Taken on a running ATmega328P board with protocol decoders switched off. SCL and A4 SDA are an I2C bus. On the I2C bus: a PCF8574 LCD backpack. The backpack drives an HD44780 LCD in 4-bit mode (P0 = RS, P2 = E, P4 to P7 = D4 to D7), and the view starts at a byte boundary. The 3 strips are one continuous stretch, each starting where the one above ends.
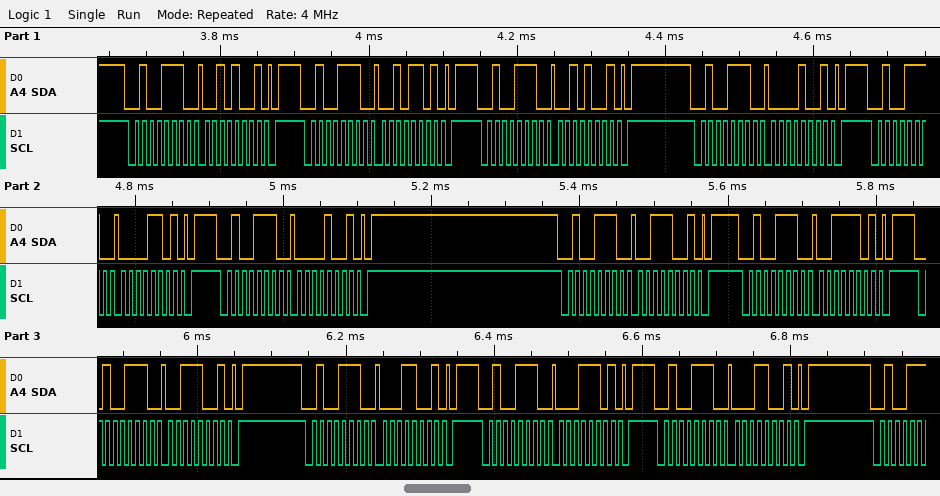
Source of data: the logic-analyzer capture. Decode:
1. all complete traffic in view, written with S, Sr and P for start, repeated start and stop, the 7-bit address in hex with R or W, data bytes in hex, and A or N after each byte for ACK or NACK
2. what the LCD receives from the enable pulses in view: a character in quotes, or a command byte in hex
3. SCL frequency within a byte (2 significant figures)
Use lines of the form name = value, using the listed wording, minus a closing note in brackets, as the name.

all complete traffic in view, written with S, Sr and P for start, repeated start and stop, the 7-bit address in hex with R or W, data bytes in hex, and A or N after each byte for ACK or NACK = S 27W A 29 A P S 27W A 2D A P S 27W A 29 A P S 27W A 09 A P S 27W A 0D A P S 27W A 09 A P S 27W A 39 A P S 27W A 3D A P S 27W A 39 A P S 27W A 19 A P S 27W A 1D A P S 27W A 19 A P
what the LCD receives from the enable pulses in view: a character in quotes, or a command byte in hex = ' ' '1'
SCL frequency within a byte = 100 kHz
